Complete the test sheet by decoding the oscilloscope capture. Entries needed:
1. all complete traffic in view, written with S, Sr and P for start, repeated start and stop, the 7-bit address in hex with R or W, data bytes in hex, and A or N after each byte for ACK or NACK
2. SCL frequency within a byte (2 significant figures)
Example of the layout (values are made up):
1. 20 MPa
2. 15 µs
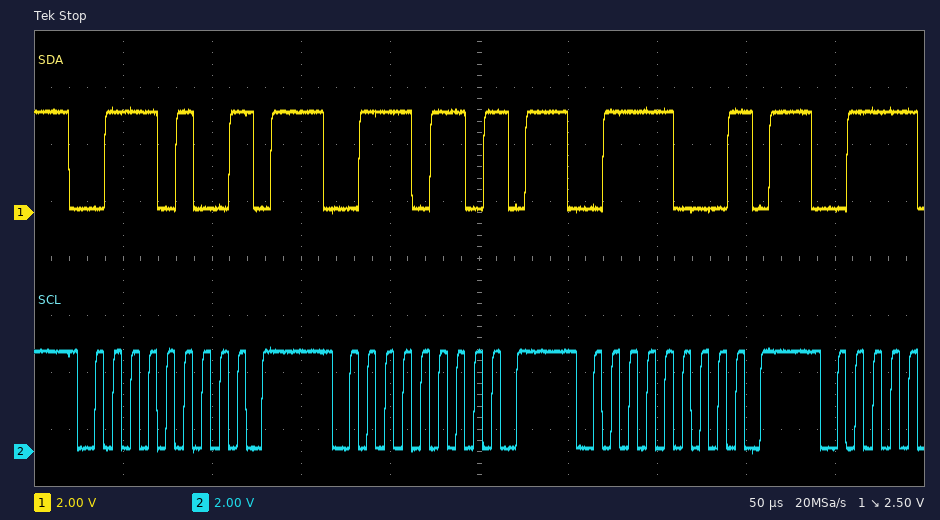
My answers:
1. S 3AW N P S 3BW N P S 3CW N P
2. 100 kHz
